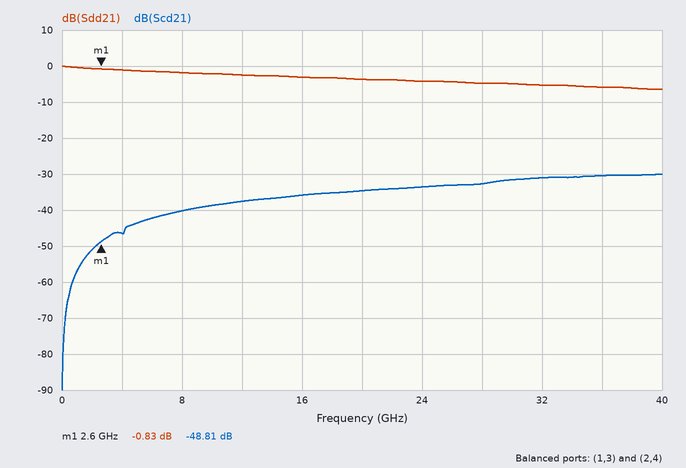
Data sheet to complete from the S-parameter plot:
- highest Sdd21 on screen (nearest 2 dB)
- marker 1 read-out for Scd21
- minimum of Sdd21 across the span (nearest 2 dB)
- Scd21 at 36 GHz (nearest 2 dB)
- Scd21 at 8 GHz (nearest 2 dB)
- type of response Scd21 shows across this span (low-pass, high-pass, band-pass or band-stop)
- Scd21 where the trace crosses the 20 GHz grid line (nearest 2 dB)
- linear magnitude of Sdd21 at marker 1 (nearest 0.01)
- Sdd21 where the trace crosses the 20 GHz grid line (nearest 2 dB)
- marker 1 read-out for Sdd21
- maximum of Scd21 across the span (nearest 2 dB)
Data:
0 dB
-48.81 dB
-6 dB
-30 dB
-40 dB
high-pass
-34 dB
0.91
-4 dB
-0.83 dB
-30 dB
